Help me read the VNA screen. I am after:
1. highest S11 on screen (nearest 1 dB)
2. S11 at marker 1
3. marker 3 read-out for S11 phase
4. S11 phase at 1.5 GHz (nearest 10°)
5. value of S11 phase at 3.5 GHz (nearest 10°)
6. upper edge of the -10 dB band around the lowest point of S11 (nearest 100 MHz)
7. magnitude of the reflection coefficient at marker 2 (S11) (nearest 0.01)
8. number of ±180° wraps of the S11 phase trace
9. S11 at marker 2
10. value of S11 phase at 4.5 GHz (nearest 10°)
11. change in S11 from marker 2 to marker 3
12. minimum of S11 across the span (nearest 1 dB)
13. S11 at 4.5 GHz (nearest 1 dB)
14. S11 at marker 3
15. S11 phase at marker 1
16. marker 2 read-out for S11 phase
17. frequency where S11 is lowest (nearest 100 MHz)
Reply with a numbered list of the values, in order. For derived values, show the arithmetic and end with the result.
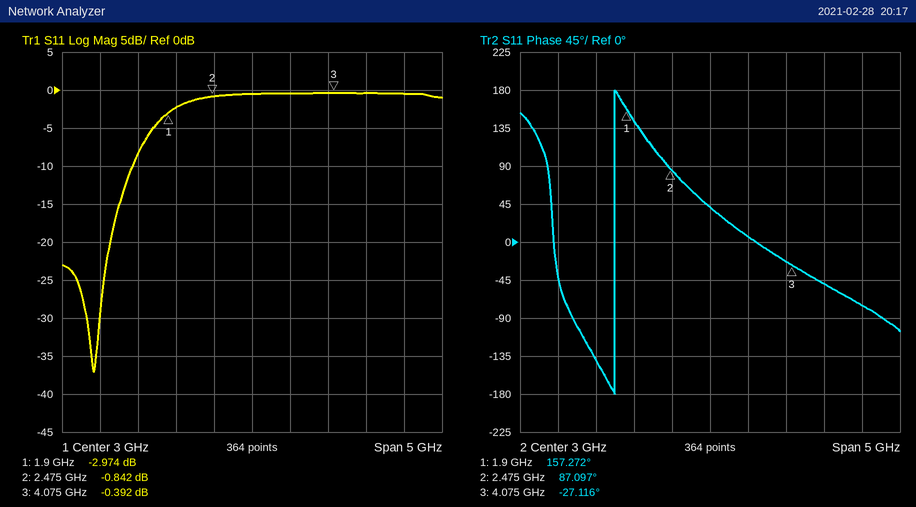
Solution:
1. 0 dB
2. -2.974 dB
3. -27.116°
4. -140°
5. 10°
6. 1.4 GHz
7. 10^(-0.842/20) ≈ 0.91
8. 1
9. -0.842 dB
10. -50°
11. -0.392 − (-0.842) = 0.450 dB
12. -37 dB
13. 0 dB
14. -0.392 dB
15. 157.272°
16. 87.097°
17. 900 MHz
